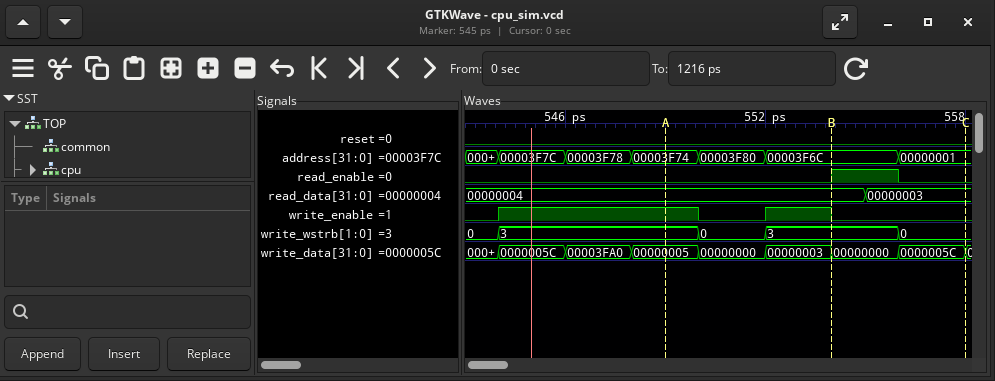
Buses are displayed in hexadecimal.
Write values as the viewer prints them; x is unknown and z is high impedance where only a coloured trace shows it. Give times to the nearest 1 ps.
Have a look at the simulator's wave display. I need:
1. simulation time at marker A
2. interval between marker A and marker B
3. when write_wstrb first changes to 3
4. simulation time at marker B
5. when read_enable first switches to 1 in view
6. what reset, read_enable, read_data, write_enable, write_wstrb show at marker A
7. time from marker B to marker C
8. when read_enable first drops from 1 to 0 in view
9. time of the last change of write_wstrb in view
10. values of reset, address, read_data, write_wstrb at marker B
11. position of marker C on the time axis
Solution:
549 ps
5 ps
544 ps
554 ps
554 ps
reset=0, read_enable=0, read_data=00000004, write_enable=1, write_wstrb=3
4 ps
556 ps
556 ps
reset=0, address=00003F6C, read_data=00000004, write_wstrb=3
558 ps
